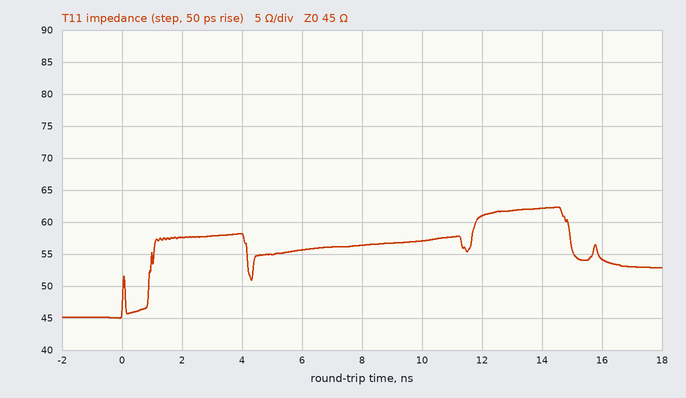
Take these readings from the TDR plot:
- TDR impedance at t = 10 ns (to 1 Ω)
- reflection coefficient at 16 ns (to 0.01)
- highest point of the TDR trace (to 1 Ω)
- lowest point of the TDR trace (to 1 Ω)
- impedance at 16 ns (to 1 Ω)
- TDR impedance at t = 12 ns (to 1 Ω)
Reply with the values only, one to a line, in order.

57 Ω
+0.09
62 Ω
45 Ω
54 Ω
61 Ω
